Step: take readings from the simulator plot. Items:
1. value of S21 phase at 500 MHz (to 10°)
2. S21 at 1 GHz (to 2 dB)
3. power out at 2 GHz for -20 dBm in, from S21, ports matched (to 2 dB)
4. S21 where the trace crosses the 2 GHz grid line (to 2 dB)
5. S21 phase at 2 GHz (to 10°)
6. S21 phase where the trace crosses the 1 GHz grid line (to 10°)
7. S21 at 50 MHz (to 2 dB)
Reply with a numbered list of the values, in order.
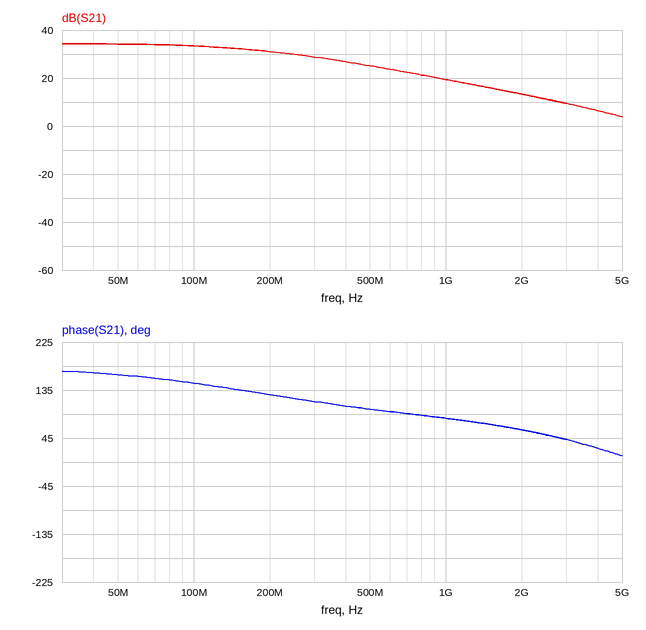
1. 100°
2. 20 dB
3. -6 dBm
4. 14 dB
5. 60°
6. 80°
7. 34 dB
